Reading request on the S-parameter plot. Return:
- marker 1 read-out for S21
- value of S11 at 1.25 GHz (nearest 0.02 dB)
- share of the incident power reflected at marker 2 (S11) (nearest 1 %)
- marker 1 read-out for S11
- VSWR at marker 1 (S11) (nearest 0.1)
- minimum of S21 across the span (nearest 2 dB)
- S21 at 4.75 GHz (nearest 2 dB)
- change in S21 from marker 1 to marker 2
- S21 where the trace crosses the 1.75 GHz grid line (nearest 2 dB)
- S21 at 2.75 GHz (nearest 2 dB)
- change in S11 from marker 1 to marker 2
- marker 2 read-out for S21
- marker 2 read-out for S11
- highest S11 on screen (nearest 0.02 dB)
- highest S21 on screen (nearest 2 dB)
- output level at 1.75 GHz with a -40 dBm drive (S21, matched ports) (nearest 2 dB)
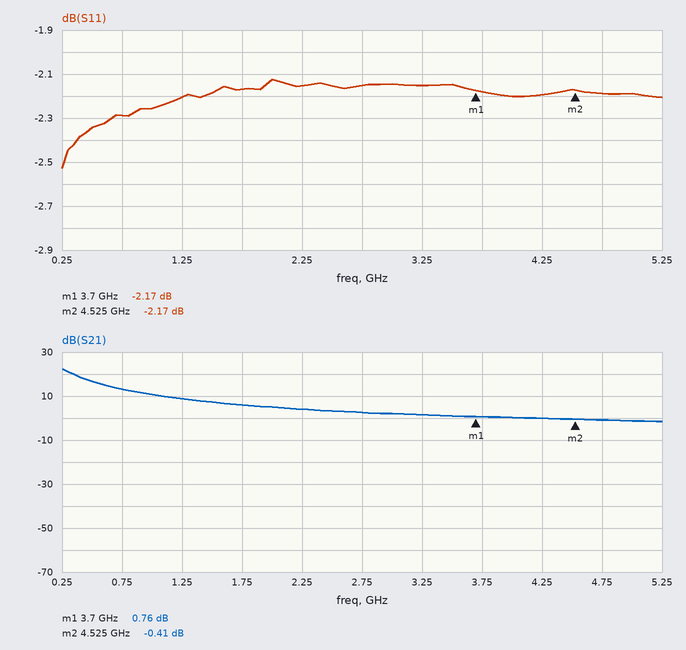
0.76 dB
-2.20 dB
61 %
-2.17 dB
8.0
-2 dB
0 dB
-1.17 dB
6 dB
2 dB
0.00 dB
-0.41 dB
-2.17 dB
-2.12 dB
22 dB
-34 dBm
